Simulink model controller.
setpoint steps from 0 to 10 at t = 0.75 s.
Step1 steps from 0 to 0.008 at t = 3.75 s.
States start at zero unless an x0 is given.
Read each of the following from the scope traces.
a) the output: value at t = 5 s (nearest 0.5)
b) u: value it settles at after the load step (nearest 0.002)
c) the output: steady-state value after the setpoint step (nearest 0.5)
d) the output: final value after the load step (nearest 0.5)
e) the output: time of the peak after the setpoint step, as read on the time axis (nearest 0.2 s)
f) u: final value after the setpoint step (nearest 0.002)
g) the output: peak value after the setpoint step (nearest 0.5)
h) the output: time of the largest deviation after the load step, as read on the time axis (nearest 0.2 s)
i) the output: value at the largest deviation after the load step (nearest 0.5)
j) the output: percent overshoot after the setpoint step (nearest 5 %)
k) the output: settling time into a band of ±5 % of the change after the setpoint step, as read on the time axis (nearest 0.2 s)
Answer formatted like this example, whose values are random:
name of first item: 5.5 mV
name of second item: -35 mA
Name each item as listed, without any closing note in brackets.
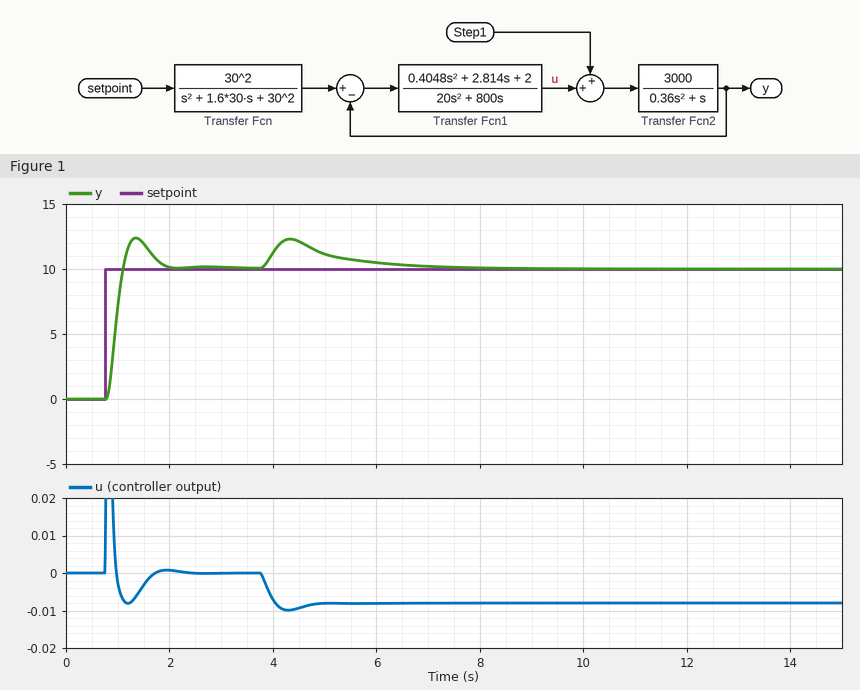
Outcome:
the output: value at t = 5 s: 11.0
u: value it settles at after the load step: -0.008
the output: steady-state value after the setpoint step: 10.0
the output: final value after the load step: 10.0
the output: time of the peak after the setpoint step, as read on the time axis: 1.4 s
u: final value after the setpoint step: 0.000
the output: peak value after the setpoint step: 12.5
the output: time of the largest deviation after the load step, as read on the time axis: 4.4 s
the output: value at the largest deviation after the load step: 12.5
the output: percent overshoot after the setpoint step: 25 %
the output: settling time into a band of ±5 % of the change after the setpoint step, as read on the time axis: 1.8 s
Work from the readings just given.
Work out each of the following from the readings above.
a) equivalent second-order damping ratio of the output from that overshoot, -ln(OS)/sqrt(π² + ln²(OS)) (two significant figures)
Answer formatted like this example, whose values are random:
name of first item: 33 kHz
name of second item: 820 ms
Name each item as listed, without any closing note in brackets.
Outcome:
equivalent second-order damping ratio of the output from that overshoot, -ln(OS)/sqrt(π² + ln²(OS)): 0.40
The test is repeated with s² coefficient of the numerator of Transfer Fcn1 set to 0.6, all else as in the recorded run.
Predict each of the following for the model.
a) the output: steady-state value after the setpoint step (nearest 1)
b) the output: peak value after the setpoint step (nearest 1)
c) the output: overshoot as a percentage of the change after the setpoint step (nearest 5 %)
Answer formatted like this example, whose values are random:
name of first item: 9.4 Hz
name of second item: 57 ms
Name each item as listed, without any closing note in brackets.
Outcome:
the output: steady-state value after the setpoint step: 10
the output: peak value after the setpoint step: 11
the output: overshoot as a percentage of the change after the setpoint step: 15 %
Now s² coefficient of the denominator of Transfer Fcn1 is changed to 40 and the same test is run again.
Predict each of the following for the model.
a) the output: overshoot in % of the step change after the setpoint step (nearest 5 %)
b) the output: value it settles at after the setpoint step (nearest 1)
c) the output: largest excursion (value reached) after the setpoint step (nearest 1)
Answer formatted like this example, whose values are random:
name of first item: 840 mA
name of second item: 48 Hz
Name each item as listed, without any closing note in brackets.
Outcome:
the output: overshoot in % of the step change after the setpoint step: 30 %
the output: value it settles at after the setpoint step: 10
the output: largest excursion (value reached) after the setpoint step: 13
